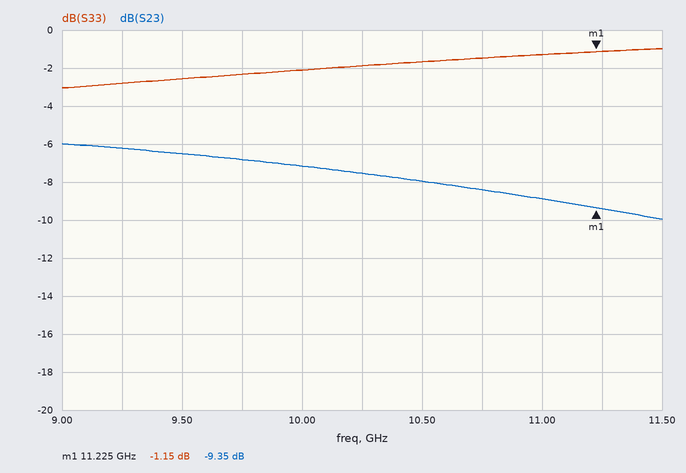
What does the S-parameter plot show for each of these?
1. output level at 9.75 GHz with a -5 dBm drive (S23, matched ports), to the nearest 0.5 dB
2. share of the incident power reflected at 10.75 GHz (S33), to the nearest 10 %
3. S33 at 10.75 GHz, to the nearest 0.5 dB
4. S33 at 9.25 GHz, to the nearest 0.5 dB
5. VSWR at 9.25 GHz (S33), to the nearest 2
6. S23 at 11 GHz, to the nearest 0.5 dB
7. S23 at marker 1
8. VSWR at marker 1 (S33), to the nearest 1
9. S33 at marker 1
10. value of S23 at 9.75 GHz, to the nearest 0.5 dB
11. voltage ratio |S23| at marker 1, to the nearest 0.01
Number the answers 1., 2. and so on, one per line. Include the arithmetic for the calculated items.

1. -5 dBm + (-7.0 dB) = -12.0 dBm
2. 10^(-1.5/10) ≈ 70.8 %, so 70 % to the nearest 10 %
3. -1.5 dB
4. -3.0 dB
5. |Γ| = 10^(-3/20) = 0.7079; VSWR = (1 + 0.7079)/(1 − 0.7079) ≈ 6
6. -9.0 dB
7. -9.35 dB
8. (1 + 0.8760)/(1 − 0.8760) ≈ 15
9. -1.15 dB
10. -7.0 dB
11. 10^(-9.35/20) ≈ 0.34
